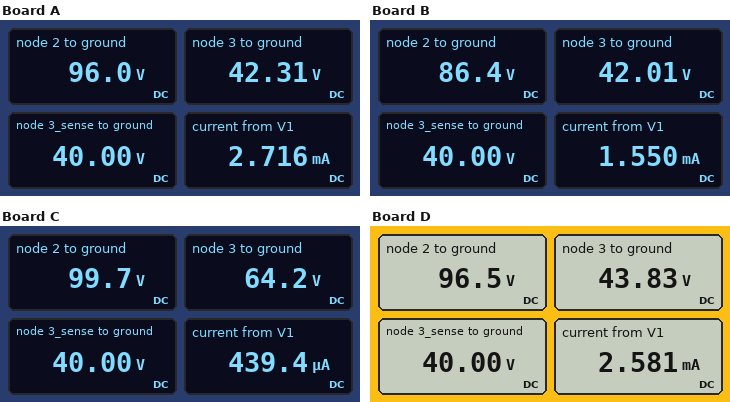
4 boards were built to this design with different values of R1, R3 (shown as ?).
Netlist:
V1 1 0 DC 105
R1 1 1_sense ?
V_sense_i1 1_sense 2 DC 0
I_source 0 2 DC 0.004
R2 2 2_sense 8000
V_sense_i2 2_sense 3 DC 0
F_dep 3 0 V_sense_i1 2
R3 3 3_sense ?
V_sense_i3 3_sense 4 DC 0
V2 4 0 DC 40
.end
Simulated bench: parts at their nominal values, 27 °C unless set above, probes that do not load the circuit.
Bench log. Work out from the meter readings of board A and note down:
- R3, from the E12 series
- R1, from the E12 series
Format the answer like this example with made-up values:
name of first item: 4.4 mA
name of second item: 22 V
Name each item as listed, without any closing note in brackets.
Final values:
R3, from the E12 series: 1.8 kΩ
R1, from the E12 series: 3.3 kΩ
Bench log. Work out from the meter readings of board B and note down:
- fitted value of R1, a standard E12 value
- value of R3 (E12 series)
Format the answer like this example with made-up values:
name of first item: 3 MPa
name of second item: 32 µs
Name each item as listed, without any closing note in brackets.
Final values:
fitted value of R1, a standard E12 value: 12 kΩ
value of R3: 820 Ω
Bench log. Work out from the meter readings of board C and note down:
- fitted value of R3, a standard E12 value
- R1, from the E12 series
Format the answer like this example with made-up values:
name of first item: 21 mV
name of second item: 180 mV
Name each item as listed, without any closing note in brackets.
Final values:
fitted value of R3, a standard E12 value: 6.8 kΩ
R1, from the E12 series: 12 kΩ
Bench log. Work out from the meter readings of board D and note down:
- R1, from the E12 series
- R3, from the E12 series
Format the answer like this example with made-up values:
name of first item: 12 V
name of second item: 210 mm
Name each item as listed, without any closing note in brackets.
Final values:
R1, from the E12 series: 3.3 kΩ
R3, from the E12 series: 2.7 kΩ
